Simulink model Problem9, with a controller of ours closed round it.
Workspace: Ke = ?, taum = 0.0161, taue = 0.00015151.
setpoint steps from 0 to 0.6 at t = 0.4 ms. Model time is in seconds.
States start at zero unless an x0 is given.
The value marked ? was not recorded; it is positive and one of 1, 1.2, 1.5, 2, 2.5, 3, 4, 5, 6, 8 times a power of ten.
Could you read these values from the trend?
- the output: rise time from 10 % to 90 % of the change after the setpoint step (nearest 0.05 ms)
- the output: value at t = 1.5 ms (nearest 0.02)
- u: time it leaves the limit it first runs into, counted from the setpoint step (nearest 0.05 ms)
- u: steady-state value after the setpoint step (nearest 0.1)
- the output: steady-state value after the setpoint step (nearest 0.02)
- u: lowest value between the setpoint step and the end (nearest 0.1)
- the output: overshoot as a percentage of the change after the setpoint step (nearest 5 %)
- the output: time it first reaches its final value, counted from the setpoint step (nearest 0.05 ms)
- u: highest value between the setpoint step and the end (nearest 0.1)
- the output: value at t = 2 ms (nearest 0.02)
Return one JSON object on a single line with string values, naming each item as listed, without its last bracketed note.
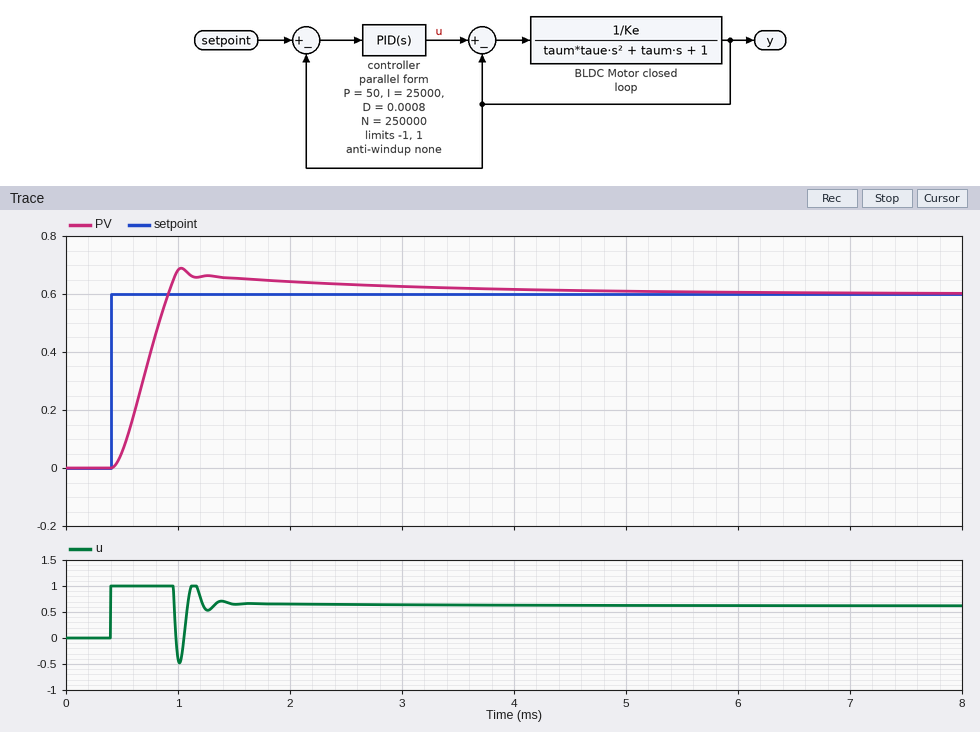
{"the output: rise time from 10 % to 90 % of the change after the setpoint step": "0.35 ms", "the output: value at t = 1.5 ms": "0.66", "u: time it leaves the limit it first runs into, counted from the setpoint step": "0.55 ms", "u: steady-state value after the setpoint step": "0.6", "the output: steady-state value after the setpoint step": "0.60", "u: lowest value between the setpoint step and the end": "-0.5", "the output: overshoot as a percentage of the change after the setpoint step": "15 %", "the output: time it first reaches its final value, counted from the setpoint step": "0.50 ms", "u: highest value between the setpoint step and the end": "1.0", "the output: value at t = 2 ms": "0.64"}
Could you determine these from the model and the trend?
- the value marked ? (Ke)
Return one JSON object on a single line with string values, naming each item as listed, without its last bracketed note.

{"the value marked ?": "0.03"}
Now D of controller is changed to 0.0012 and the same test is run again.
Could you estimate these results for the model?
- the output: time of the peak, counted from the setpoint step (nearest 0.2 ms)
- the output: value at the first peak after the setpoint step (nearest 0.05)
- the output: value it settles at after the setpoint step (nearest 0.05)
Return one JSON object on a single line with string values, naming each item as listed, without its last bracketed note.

{"the output: time of the peak, counted from the setpoint step": "0.6 ms", "the output: value at the first peak after the setpoint step": "0.70", "the output: value it settles at after the setpoint step": "0.60"}
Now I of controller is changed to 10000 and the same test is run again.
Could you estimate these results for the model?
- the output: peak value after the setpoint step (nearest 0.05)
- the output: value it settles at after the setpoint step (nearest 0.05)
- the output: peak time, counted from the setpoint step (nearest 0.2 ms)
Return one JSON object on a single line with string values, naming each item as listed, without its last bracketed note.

{"the output: peak value after the setpoint step": "0.65", "the output: value it settles at after the setpoint step": "0.60", "the output: peak time, counted from the setpoint step": "0.6 ms"}
